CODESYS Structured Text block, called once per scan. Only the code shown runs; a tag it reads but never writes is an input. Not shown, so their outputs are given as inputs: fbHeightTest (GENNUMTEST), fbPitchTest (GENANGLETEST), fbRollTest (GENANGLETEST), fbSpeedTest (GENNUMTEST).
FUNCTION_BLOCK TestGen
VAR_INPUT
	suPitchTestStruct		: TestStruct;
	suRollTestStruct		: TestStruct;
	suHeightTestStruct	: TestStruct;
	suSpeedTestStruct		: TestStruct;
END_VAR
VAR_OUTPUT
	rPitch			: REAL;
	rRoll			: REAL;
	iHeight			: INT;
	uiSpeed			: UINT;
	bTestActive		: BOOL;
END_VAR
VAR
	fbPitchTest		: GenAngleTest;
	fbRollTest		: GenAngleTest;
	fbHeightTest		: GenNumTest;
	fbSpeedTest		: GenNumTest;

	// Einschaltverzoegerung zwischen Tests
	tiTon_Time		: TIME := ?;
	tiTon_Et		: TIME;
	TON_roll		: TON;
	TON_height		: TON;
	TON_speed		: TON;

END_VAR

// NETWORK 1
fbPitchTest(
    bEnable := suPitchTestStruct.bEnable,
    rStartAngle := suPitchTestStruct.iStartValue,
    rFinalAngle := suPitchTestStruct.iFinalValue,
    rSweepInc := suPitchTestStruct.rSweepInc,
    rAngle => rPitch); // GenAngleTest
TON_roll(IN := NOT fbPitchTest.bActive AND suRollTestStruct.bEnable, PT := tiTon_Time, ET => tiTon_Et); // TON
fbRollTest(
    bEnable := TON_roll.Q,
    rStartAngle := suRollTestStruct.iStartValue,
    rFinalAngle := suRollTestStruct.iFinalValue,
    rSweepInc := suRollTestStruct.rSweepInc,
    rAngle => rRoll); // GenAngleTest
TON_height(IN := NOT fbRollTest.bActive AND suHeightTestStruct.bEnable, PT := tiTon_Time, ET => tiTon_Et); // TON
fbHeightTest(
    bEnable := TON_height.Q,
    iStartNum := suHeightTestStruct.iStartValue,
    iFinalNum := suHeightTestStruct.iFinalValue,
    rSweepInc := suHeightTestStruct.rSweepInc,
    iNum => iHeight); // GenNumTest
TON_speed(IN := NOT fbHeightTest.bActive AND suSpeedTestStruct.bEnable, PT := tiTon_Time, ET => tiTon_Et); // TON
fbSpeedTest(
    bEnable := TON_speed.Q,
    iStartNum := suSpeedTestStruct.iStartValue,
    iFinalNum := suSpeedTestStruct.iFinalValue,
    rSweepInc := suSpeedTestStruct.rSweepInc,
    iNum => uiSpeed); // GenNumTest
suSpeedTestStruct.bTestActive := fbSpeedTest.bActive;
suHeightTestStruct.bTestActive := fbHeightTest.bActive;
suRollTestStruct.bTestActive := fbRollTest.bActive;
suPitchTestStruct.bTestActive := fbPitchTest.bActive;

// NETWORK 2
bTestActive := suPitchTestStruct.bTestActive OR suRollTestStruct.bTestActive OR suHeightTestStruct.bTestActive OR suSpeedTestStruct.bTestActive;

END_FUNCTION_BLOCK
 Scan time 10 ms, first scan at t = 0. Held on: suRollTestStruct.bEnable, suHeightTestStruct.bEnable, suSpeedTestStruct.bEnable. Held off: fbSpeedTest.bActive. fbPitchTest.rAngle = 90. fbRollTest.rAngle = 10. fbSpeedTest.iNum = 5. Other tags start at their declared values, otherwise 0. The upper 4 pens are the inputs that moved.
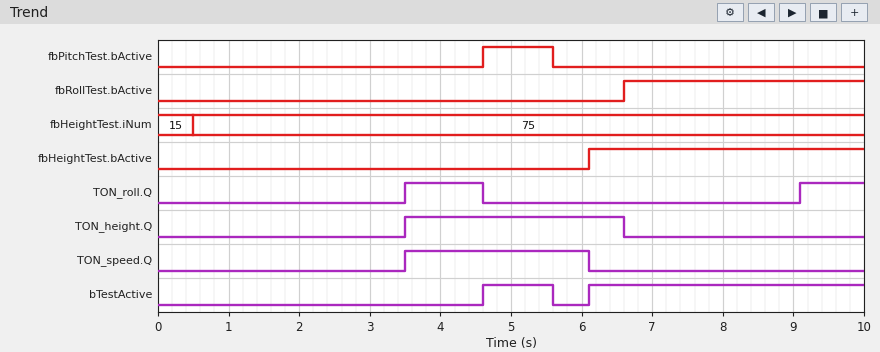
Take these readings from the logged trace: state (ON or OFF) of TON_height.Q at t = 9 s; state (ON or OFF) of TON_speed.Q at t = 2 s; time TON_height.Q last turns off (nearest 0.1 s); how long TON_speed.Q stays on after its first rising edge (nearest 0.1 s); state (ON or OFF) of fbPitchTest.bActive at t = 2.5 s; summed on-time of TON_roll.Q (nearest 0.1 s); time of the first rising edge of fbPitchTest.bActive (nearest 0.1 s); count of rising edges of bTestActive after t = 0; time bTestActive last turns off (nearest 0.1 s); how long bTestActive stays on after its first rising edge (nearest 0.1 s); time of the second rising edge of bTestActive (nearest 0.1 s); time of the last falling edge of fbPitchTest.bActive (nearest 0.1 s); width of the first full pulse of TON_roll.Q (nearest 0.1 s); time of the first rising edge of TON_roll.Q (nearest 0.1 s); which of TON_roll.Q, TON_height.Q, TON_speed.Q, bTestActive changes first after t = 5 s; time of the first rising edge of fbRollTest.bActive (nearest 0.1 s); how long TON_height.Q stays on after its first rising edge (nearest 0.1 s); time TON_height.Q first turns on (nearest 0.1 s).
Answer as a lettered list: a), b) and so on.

a) OFF
b) OFF
c) 6.6 s
d) 2.6 s
e) OFF
f) 2.0 s
g) 4.6 s
h) 2
i) 5.6 s
j) 1.0 s
k) 6.1 s
l) 5.6 s
m) 1.1 s
n) 3.5 s
o) bTestActive
p) 6.6 s
q) 3.1 s
r) 3.5 s
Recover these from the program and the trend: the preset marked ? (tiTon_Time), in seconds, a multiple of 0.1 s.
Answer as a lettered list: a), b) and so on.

a) 3.5 s
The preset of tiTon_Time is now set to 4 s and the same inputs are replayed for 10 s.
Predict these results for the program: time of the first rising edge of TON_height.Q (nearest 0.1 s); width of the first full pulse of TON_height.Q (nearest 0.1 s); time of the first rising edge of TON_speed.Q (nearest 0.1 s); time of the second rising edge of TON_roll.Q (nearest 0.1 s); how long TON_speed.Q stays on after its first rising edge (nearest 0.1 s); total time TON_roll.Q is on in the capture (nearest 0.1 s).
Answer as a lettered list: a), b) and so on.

a) 4.0 s
b) 2.6 s
c) 4.0 s
d) 9.6 s
e) 2.1 s
f) 1.0 s
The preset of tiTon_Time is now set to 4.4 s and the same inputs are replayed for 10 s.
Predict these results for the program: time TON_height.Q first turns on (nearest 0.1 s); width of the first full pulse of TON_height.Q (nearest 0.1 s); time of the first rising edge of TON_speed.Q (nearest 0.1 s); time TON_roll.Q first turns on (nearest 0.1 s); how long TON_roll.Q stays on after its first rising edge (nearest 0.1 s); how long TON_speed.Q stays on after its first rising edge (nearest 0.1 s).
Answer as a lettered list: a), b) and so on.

a) 4.4 s
b) 2.2 s
c) 4.4 s
d) 4.4 s
e) 0.2 s
f) 1.7 s
